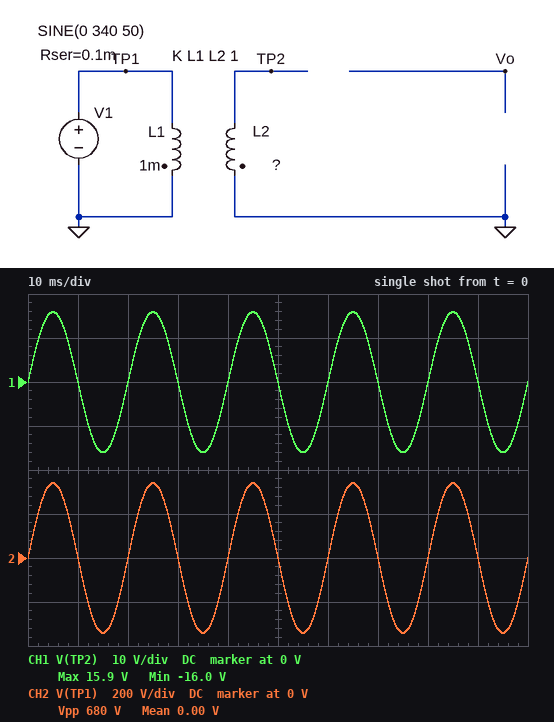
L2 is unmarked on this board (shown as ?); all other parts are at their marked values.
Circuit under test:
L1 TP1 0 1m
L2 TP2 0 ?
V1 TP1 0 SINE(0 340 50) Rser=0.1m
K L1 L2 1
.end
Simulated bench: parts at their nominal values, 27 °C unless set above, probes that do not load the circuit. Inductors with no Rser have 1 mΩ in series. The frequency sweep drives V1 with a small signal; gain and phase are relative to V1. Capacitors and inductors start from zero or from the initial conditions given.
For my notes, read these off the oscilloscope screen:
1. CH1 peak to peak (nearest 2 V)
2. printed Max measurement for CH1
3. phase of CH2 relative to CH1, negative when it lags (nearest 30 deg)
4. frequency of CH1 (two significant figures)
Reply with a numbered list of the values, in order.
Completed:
1. 32 V
2. 15.9 V
3. 0 deg
4. 50 Hz
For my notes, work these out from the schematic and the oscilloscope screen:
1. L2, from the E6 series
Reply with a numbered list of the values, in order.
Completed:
1. 2.2 µH
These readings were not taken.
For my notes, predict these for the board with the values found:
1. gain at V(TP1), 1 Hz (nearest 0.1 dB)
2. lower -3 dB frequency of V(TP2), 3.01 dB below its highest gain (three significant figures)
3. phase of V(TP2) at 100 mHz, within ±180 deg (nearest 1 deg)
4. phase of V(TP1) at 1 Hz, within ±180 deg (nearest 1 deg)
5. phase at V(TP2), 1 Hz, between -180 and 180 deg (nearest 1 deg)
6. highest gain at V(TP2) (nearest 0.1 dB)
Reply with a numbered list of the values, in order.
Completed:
1. 0 dB
2. 175 mHz
3. 60 deg
4. 1 deg
5. 10 deg
6. -26.6 dB
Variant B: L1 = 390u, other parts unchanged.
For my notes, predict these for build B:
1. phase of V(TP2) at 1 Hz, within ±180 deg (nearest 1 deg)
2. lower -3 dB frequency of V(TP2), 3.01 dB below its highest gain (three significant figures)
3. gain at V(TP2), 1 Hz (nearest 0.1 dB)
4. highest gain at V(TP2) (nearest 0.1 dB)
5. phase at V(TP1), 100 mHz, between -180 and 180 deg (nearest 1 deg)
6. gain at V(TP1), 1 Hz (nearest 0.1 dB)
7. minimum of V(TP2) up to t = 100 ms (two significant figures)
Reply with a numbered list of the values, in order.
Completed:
1. 24 deg
2. 449 mHz
3. -23.3 dB
4. -22.5 dB
5. 1 deg
6. -0.1 dB
7. -26 V
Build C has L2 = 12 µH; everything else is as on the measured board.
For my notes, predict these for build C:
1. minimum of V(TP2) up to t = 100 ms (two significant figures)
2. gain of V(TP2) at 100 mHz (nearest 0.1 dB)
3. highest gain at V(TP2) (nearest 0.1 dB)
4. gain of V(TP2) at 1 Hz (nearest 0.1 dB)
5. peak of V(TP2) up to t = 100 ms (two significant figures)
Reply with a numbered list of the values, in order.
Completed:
1. -37 V
2. -25.3 dB
3. -19.2 dB
4. -19.3 dB
5. 37 V
